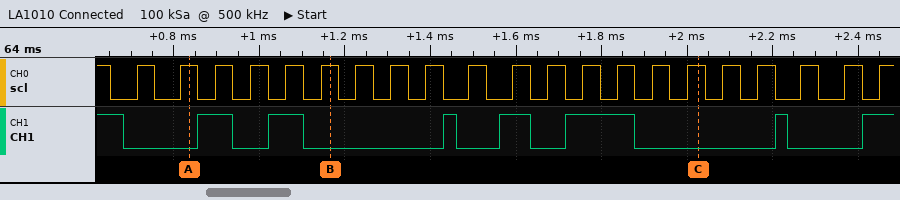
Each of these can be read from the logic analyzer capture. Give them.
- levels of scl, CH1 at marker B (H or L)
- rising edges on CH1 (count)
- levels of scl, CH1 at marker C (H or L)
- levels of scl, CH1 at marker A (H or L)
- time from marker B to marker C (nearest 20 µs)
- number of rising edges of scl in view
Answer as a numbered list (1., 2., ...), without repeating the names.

1. scl=H, CH1=L
2. 7
3. scl=H, CH1=L
4. scl=H, CH1=L
5. 860 µs
6. 21
